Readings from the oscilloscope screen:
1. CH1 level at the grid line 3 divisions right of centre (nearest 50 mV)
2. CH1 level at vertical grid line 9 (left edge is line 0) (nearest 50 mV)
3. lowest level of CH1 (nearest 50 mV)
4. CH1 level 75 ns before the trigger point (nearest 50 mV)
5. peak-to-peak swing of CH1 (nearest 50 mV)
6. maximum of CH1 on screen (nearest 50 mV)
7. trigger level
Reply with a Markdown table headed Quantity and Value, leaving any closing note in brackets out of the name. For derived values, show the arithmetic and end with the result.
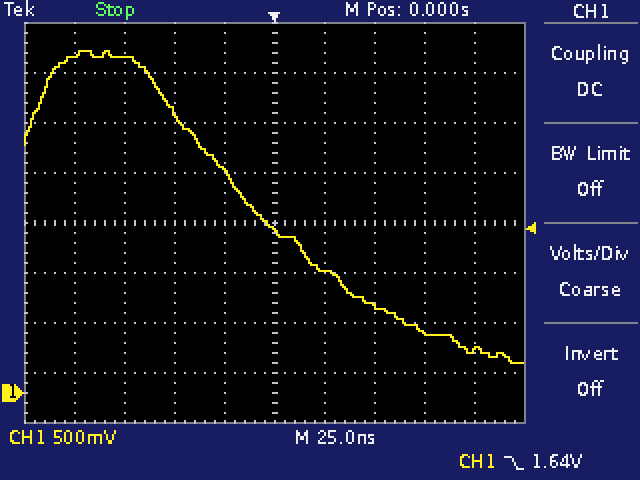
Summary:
| Quantity | Value |
|---|---|
| CH1 level at the grid line 3 divisions right of centre | 600 mV |
| CH1 level at vertical grid line 9 (left edge is line 0) | 450 mV |
| lowest level of CH1 | 300 mV |
| CH1 level 75 ns before the trigger point | 3.35 V |
| peak-to-peak swing of CH1 | 3.40 V − (300 mV) = 3.10 V |
| maximum of CH1 on screen | 3.40 V |
| trigger level | 1.64 V |
